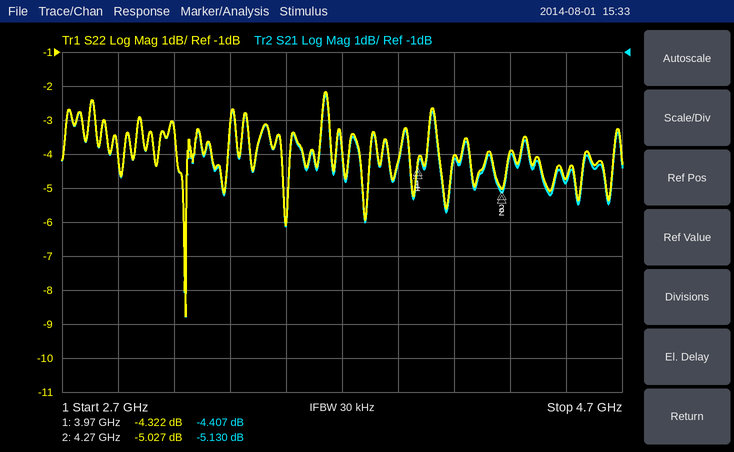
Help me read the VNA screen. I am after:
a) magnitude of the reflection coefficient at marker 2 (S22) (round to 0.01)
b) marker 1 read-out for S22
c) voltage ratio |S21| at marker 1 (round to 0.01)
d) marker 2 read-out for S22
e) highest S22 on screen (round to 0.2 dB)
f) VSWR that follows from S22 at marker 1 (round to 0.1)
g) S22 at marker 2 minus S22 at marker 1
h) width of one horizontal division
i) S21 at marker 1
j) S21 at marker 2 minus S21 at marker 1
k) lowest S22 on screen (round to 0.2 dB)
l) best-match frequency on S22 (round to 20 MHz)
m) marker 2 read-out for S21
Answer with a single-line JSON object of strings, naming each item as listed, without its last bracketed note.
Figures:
{"magnitude of the reflection coefficient at marker 2 (S22)": "0.56", "marker 1 read-out for S22": "-4.322 dB", "voltage ratio |S21| at marker 1": "0.60", "marker 2 read-out for S22": "-5.027 dB", "highest S22 on screen": "-2.2 dB", "VSWR that follows from S22 at marker 1": "4.1", "S22 at marker 2 minus S22 at marker 1": "-0.705 dB", "width of one horizontal division": "200 MHz", "S21 at marker 1": "-4.407 dB", "S21 at marker 2 minus S21 at marker 1": "-0.723 dB", "lowest S22 on screen": "-8.8 dB", "best-match frequency on S22": "3.14 GHz", "marker 2 read-out for S21": "-5.130 dB"}
